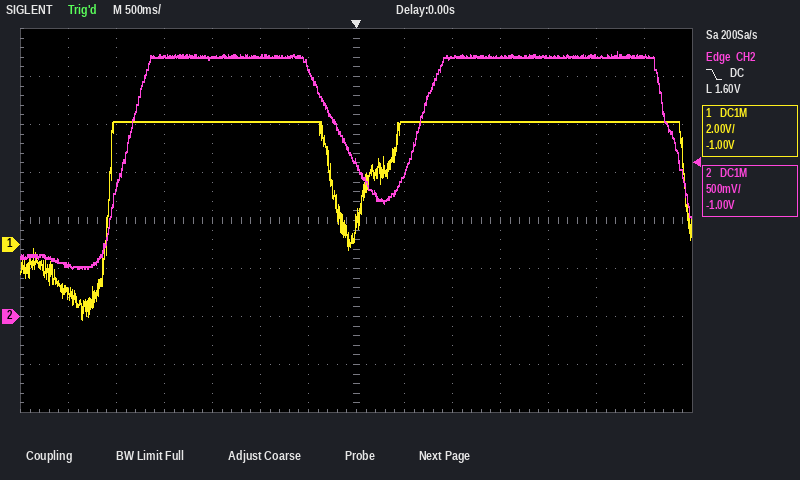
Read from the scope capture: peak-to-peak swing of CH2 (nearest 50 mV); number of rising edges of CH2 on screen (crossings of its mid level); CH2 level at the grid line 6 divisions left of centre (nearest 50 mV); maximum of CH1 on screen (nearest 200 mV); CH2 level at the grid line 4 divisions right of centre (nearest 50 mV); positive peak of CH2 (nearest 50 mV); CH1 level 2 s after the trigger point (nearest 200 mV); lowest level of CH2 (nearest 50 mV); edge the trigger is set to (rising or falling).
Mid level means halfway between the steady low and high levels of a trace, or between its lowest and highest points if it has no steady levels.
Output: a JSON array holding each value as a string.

["2.25 V", "2", "550 mV", "5.2 V", "2.70 V", "2.75 V", "5.2 V", "500 mV", "falling"]
